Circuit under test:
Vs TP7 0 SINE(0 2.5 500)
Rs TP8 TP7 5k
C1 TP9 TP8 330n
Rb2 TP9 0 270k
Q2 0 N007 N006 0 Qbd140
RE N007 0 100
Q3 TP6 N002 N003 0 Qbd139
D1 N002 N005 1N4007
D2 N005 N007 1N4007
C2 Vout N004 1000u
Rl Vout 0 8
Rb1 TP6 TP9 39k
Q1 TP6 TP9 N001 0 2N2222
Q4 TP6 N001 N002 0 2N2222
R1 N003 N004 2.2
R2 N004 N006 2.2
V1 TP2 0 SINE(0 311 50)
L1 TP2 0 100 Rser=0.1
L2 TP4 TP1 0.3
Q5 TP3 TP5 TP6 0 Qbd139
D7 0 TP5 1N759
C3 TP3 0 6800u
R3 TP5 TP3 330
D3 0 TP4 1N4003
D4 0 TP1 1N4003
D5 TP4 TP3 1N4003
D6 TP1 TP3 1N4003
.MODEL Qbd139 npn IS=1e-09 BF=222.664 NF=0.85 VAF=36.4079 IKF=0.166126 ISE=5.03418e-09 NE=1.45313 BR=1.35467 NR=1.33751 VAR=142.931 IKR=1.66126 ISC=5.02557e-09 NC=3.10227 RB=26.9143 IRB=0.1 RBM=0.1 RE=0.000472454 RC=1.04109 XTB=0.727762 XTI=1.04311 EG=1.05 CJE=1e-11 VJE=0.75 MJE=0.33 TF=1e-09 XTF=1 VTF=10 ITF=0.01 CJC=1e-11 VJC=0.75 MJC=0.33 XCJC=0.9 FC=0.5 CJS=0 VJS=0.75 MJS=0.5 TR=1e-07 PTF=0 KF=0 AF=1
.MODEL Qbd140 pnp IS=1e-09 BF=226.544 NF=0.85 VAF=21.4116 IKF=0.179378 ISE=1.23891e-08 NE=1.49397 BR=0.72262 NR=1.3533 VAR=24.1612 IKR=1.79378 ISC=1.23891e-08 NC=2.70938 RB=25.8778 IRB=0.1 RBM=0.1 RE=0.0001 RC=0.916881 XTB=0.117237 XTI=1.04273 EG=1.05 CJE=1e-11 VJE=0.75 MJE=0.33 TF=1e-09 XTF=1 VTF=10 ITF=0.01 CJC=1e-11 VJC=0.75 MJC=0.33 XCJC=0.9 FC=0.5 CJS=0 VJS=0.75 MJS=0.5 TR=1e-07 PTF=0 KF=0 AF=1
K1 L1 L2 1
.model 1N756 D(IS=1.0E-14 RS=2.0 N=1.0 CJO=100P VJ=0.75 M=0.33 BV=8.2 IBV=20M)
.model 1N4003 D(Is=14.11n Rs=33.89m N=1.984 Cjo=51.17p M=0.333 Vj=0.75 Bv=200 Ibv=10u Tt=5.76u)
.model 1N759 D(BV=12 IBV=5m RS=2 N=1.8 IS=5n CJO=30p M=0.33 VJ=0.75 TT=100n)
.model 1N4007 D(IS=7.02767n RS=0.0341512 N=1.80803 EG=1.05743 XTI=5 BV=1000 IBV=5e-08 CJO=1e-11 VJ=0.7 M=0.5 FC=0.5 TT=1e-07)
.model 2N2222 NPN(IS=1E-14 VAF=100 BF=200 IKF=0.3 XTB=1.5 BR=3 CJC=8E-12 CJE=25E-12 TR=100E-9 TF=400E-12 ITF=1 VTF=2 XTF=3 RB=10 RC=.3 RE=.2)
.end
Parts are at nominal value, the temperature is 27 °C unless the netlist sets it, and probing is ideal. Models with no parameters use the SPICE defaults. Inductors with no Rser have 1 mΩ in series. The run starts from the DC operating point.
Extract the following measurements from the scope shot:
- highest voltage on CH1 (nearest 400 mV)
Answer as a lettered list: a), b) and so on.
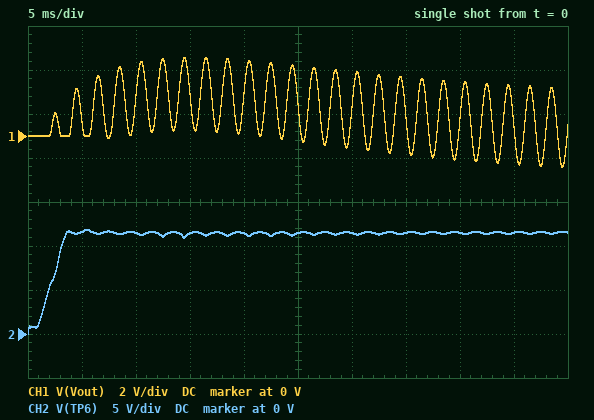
a) 3.6 V
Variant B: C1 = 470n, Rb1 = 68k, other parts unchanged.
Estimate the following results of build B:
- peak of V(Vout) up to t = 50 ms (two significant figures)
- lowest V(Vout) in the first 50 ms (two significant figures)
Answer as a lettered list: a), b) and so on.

a) 2.8 V
b) -1.3 V
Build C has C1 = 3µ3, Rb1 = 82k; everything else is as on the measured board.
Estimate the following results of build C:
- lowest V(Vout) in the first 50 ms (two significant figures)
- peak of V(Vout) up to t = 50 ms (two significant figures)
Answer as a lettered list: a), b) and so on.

a) -420 mV
b) 1.3 V
